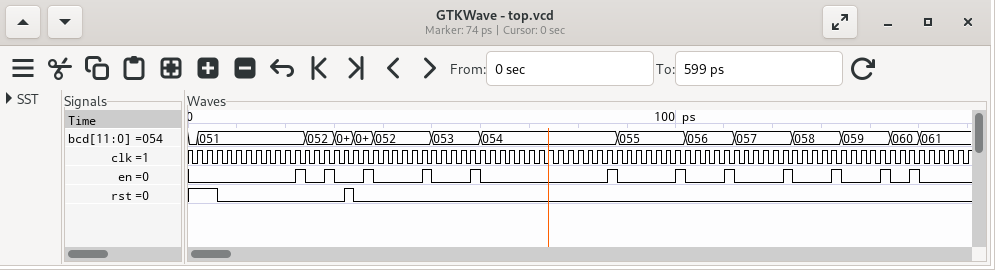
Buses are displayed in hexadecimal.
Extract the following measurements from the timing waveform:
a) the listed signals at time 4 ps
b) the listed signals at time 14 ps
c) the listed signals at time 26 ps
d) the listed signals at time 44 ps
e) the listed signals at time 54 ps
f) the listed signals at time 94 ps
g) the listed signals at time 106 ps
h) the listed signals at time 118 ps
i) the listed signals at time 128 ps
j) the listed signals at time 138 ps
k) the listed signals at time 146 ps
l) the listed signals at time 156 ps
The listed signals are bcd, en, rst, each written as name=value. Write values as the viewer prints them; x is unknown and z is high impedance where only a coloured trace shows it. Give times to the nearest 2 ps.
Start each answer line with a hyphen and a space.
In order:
- bcd=051, en=0, rst=1
- bcd=051, en=0, rst=0
- bcd=052, en=0, rst=0
- bcd=052, en=0, rst=0
- bcd=053, en=0, rst=0
- bcd=055, en=0, rst=0
- bcd=056, en=0, rst=0
- bcd=057, en=0, rst=0
- bcd=058, en=0, rst=0
- bcd=059, en=0, rst=0
- bcd=060, en=0, rst=0
- bcd=061, en=0, rst=0
